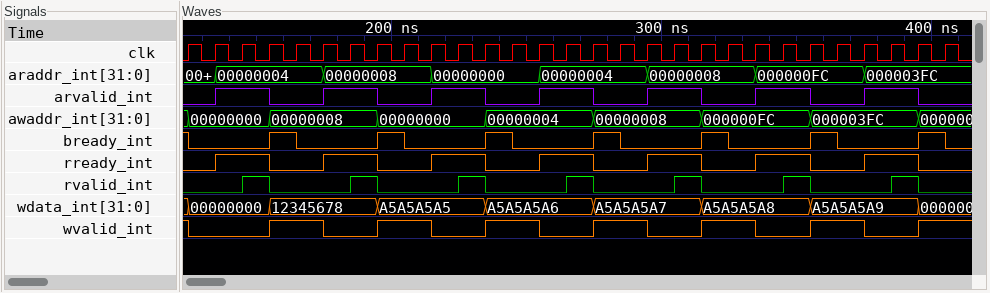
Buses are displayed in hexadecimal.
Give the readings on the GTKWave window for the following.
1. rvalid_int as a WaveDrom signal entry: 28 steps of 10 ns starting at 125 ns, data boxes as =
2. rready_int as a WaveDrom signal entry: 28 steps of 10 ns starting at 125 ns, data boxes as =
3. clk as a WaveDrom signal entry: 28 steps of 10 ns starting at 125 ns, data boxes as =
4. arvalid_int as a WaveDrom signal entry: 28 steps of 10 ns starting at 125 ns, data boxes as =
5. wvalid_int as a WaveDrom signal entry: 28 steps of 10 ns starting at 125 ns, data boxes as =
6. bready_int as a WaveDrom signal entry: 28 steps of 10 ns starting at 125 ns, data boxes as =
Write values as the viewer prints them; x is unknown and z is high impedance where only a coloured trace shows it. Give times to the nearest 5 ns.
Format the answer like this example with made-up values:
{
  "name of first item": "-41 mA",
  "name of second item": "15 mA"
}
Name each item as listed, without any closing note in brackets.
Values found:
{
  "rvalid_int as a WaveDrom signal entry: 28 steps of 10 ns starting at 125 ns, data boxes as =": "{name: 'rvalid_int', wave: '0.10..10..10..10..10..10..10'}",
  "rready_int as a WaveDrom signal entry: 28 steps of 10 ns starting at 125 ns, data boxes as =": "{name: 'rready_int', wave: '01.0.1.0.1.0.1.0.1.0.1.0.1.0'}",
  "clk as a WaveDrom signal entry: 28 steps of 10 ns starting at 125 ns, data boxes as =": "{name: 'clk', wave: 'p...........................'}",
  "arvalid_int as a WaveDrom signal entry: 28 steps of 10 ns starting at 125 ns, data boxes as =": "{name: 'arvalid_int', wave: '01.0.1.0.1.0.1.0.1.0.1.0.1.0'}",
  "wvalid_int as a WaveDrom signal entry: 28 steps of 10 ns starting at 125 ns, data boxes as =": "{name: 'wvalid_int', wave: '0..1.0.1.0.1.0.1.0.1.0.1.0.1'}",
  "bready_int as a WaveDrom signal entry: 28 steps of 10 ns starting at 125 ns, data boxes as =": "{name: 'bready_int', wave: '0..10..10..10..10..10..10..1'}"
}
